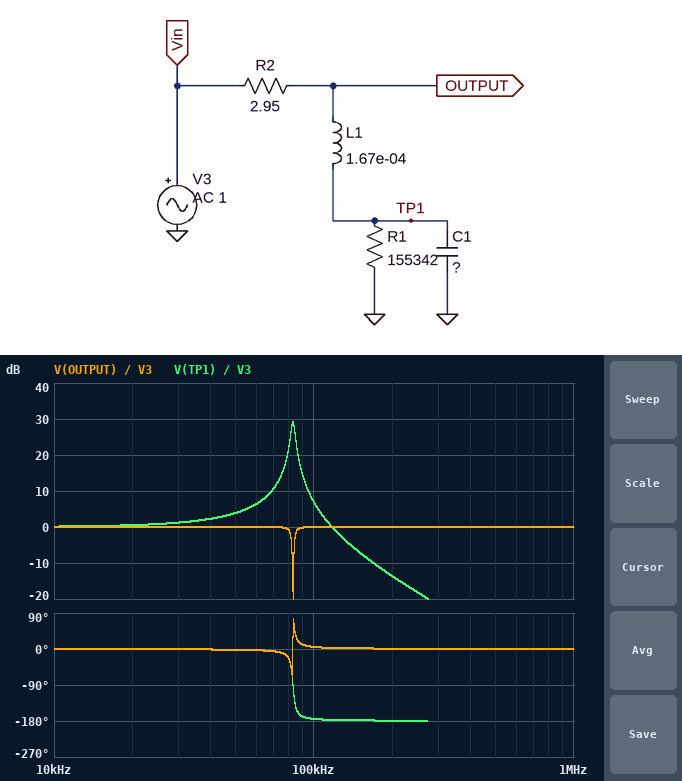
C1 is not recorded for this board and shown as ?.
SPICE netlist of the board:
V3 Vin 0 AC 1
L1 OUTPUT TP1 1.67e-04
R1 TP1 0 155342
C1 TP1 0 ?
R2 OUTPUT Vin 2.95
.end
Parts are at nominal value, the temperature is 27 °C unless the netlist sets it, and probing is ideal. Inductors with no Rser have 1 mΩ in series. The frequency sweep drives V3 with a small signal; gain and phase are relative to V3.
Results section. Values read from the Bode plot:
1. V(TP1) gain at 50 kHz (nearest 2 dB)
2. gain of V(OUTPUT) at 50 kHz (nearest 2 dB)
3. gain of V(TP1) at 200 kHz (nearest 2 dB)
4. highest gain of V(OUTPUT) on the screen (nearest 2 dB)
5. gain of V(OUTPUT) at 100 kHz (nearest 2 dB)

4 dB
0 dB
-14 dB
0 dB
0 dB
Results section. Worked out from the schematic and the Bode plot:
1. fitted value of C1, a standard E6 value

22 nF
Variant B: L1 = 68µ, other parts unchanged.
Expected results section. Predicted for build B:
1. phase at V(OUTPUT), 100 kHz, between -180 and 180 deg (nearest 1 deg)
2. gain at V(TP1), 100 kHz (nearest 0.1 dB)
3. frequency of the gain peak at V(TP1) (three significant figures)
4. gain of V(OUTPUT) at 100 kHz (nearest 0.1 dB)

-6 deg
7.7 dB
130 kHz
0 dB
